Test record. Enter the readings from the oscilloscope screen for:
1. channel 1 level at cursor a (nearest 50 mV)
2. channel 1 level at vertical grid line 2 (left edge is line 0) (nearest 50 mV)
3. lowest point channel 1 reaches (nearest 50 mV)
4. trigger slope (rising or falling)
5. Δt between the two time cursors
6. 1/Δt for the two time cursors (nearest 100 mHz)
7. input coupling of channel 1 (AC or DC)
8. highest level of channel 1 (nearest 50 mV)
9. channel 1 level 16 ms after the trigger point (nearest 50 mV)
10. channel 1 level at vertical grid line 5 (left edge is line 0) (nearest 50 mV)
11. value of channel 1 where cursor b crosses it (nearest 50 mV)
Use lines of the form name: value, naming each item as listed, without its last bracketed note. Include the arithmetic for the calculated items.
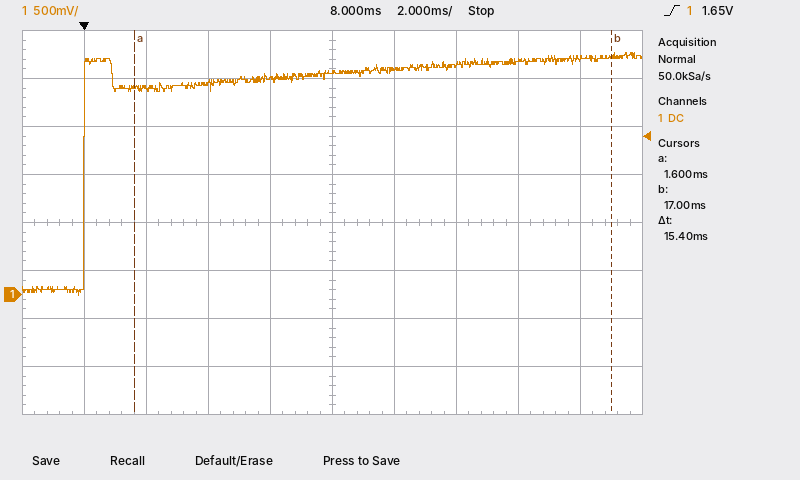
channel 1 level at cursor a: 2.15 V
channel 1 level at vertical grid line 2 (left edge is line 0): 2.15 V
lowest point channel 1 reaches: 0 mV
trigger slope: rising
Δt between the two time cursors: 15.4 ms
1/Δt for the two time cursors: 1 / 15.4 ms ≈ 64.9 Hz
input coupling of channel 1: DC
highest level of channel 1: 2.50 V
channel 1 level 16 ms after the trigger point: 2.45 V
channel 1 level at vertical grid line 5 (left edge is line 0): 2.30 V
value of channel 1 where cursor b crosses it: 2.50 V
